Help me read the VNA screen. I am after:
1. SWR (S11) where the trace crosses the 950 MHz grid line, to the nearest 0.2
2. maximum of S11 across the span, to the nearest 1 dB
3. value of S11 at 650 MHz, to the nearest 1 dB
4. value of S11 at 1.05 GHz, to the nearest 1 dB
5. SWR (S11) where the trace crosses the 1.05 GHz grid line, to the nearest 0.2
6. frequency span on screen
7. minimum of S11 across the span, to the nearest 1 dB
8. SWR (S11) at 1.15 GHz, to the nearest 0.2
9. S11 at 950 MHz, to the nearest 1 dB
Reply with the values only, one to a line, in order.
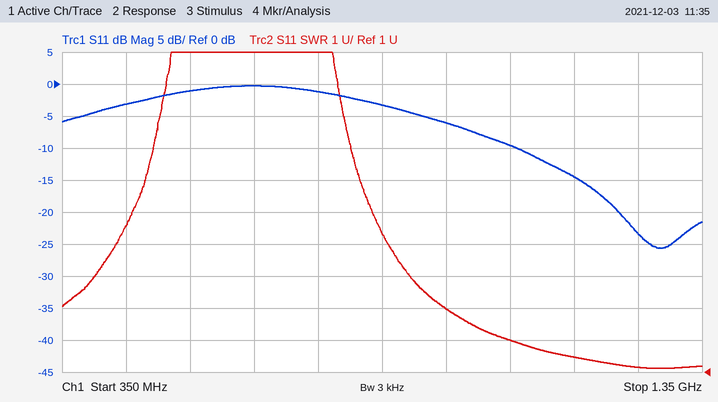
3.0
0 dB
0 dB
-10 dB
2.0
1 GHz
-26 dB
1.4
-6 dB
